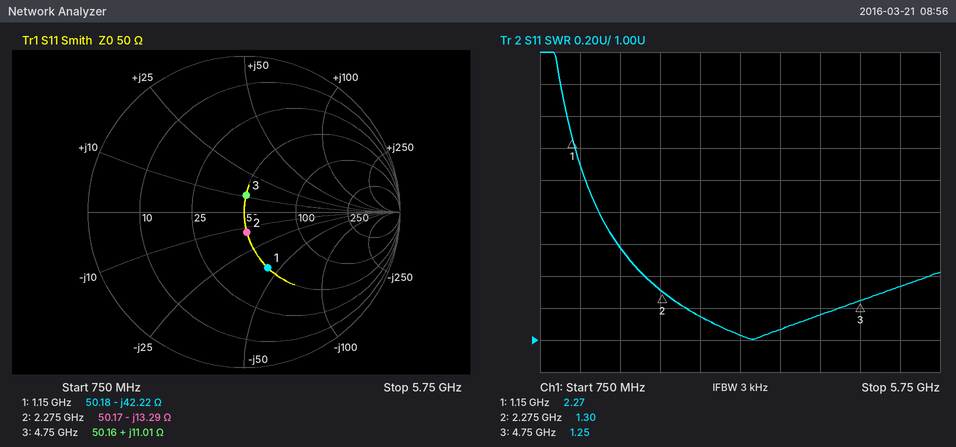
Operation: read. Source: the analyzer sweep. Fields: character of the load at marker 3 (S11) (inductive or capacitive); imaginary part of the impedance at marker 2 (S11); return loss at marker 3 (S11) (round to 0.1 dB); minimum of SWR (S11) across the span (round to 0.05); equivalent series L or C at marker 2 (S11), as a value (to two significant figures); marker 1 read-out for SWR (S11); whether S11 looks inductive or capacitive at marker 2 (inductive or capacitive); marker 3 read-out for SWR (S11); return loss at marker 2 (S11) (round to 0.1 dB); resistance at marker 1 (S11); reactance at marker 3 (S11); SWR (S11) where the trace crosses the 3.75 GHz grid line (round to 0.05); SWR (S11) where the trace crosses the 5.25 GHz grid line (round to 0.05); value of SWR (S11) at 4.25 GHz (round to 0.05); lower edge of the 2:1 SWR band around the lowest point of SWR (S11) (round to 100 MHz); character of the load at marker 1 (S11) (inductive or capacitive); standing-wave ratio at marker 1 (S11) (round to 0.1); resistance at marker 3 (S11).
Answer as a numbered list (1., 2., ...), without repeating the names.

1. inductive
2. -13.29 Ω
3. 19.2 dB
4. 1.00
5. 5.3 pF
6. 2.27
7. capacitive
8. 1.25
9. 17.6 dB
10. 50.18 Ω
11. +11.01 Ω
12. 1.05
13. 1.35
14. 1.15
15. 1.3 GHz
16. capacitive
17. 2.3
18. 50.16 Ω
